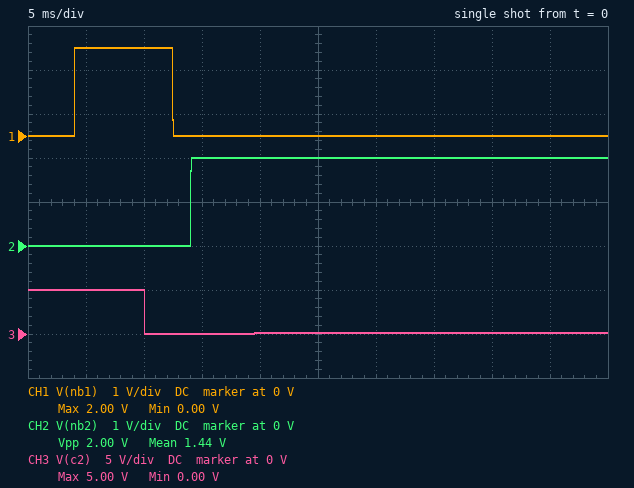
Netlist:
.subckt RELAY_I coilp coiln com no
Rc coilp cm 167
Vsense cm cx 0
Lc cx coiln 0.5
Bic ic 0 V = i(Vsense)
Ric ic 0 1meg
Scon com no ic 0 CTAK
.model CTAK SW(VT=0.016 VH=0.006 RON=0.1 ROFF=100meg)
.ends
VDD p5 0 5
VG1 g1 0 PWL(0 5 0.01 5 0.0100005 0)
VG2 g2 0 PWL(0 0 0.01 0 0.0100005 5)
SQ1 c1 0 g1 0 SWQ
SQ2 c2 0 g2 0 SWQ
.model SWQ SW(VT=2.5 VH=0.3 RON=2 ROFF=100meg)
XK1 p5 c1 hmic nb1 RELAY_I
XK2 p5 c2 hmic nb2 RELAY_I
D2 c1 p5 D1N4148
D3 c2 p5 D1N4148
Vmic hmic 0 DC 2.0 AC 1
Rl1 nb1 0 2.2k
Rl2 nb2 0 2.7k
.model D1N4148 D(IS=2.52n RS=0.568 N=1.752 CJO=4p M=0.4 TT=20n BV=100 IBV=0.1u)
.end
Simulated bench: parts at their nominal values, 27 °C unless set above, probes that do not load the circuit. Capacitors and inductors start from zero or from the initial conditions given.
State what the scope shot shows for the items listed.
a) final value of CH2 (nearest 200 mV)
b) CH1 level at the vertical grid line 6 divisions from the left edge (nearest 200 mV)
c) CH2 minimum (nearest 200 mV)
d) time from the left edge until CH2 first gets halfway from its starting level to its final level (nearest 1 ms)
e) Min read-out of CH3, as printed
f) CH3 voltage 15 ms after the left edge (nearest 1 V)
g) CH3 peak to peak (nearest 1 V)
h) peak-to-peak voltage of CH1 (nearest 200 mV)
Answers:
2.0 V
0 V
0 V
14 ms
0.00 V
0 V
5 V
2.0 V
